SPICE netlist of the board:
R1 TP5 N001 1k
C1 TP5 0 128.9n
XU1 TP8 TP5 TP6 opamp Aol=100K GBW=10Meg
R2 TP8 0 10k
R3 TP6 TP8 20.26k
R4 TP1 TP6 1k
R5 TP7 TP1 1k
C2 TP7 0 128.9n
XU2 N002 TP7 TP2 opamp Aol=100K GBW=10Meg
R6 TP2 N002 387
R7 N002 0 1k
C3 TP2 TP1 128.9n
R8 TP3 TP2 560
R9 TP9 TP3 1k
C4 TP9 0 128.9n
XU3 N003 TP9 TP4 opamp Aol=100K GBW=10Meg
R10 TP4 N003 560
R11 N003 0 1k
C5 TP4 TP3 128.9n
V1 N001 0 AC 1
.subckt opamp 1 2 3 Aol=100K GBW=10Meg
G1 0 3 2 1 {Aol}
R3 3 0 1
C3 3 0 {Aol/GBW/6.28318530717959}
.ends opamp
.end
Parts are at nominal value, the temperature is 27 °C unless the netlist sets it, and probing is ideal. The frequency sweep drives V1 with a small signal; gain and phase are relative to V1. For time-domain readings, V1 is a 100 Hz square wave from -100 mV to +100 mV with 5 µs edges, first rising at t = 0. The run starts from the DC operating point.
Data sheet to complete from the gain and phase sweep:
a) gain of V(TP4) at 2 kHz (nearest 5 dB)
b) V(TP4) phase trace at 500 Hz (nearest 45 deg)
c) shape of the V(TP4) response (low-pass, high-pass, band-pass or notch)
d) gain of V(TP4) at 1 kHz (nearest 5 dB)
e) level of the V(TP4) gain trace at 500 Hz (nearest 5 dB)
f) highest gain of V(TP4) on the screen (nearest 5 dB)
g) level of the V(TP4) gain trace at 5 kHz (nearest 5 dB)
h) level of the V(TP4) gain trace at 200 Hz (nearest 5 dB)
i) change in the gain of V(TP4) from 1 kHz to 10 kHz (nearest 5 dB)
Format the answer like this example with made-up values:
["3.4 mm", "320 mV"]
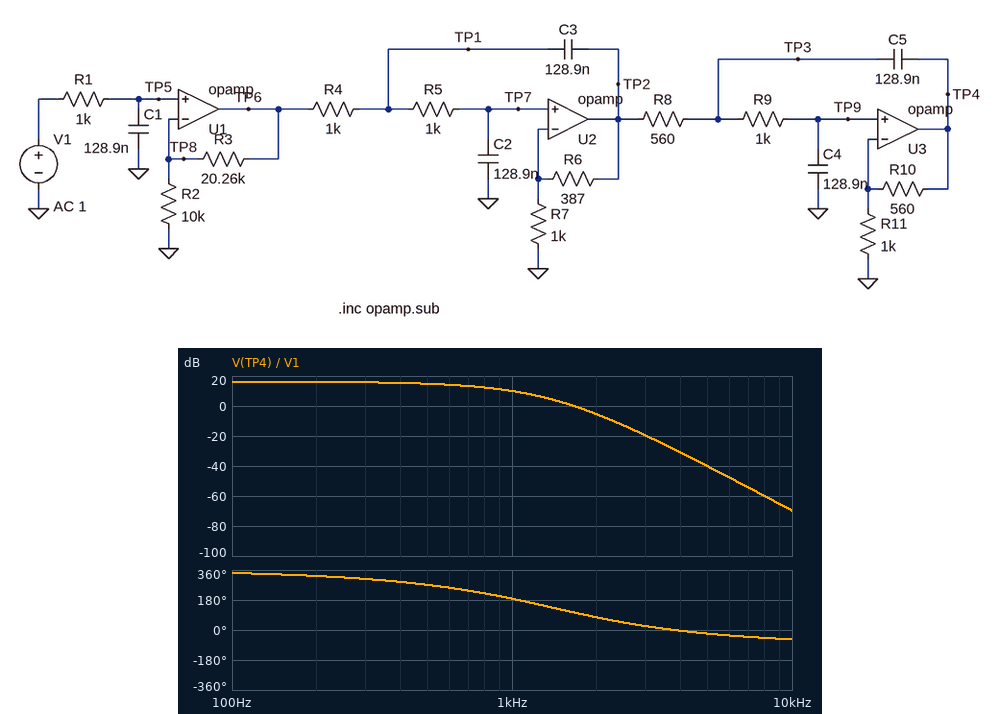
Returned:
["-5 dB", "270 deg", "low-pass", "10 dB", "15 dB", "15 dB", "-40 dB", "15 dB", "-80 dB"]
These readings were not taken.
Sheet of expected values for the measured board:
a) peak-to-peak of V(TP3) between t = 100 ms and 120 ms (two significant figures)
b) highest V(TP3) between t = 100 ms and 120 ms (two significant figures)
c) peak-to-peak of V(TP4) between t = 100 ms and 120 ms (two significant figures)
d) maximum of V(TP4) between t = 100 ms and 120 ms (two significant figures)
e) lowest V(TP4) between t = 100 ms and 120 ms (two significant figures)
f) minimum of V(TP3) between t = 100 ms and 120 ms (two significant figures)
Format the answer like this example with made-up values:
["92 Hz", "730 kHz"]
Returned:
["860 mV", "430 mV", "1.3 V", "660 mV", "-660 mV", "-430 mV"]
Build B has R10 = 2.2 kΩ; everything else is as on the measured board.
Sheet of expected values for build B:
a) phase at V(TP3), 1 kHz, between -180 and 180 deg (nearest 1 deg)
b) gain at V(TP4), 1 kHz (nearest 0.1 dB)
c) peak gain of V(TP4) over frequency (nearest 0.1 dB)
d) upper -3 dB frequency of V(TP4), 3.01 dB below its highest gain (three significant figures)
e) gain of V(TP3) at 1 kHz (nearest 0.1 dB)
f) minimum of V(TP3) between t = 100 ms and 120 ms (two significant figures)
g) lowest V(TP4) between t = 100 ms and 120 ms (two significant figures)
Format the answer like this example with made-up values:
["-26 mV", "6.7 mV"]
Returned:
["-98 deg", "21.0 dB", "22.6 dB", "1.53 kHz", "13.1 dB", "-580 mV", "-1.5 V"]
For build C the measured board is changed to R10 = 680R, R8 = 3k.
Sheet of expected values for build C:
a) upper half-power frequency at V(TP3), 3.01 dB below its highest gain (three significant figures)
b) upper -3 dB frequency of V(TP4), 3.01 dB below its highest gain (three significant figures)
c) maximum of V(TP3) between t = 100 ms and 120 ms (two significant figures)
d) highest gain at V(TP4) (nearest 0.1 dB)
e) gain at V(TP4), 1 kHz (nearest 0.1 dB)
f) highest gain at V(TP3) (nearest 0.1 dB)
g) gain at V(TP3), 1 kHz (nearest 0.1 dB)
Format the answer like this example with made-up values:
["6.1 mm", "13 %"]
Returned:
["740 Hz", "684 Hz", "510 mV", "17.0 dB", "6.8 dB", "12.8 dB", "4.5 dB"]
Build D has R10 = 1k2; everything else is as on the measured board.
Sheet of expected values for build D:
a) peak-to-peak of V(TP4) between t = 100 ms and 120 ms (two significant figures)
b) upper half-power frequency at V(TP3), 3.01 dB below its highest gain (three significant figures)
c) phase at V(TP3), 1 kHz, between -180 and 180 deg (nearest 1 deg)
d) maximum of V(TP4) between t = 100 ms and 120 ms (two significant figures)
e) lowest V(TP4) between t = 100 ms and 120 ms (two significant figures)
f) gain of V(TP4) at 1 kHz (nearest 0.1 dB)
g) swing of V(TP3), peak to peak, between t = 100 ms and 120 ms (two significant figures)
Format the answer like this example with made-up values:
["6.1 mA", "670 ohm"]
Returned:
["1.9 V", "1.11 kHz", "-124 deg", "940 mV", "-940 mV", "14.9 dB", "910 mV"]
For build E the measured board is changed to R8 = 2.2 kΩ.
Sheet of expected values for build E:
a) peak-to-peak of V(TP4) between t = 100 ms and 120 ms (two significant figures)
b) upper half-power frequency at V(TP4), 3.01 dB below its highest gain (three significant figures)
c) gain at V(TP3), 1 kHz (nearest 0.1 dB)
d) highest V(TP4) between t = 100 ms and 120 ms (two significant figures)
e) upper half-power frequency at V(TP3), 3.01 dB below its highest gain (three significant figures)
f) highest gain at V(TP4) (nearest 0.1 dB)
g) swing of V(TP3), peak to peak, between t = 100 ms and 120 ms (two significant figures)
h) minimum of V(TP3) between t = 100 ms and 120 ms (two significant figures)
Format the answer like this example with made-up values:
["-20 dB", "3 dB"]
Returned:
["1.4 V", "659 Hz", "5.5 dB", "710 mV", "752 Hz", "16.3 dB", "940 mV", "-470 mV"]
